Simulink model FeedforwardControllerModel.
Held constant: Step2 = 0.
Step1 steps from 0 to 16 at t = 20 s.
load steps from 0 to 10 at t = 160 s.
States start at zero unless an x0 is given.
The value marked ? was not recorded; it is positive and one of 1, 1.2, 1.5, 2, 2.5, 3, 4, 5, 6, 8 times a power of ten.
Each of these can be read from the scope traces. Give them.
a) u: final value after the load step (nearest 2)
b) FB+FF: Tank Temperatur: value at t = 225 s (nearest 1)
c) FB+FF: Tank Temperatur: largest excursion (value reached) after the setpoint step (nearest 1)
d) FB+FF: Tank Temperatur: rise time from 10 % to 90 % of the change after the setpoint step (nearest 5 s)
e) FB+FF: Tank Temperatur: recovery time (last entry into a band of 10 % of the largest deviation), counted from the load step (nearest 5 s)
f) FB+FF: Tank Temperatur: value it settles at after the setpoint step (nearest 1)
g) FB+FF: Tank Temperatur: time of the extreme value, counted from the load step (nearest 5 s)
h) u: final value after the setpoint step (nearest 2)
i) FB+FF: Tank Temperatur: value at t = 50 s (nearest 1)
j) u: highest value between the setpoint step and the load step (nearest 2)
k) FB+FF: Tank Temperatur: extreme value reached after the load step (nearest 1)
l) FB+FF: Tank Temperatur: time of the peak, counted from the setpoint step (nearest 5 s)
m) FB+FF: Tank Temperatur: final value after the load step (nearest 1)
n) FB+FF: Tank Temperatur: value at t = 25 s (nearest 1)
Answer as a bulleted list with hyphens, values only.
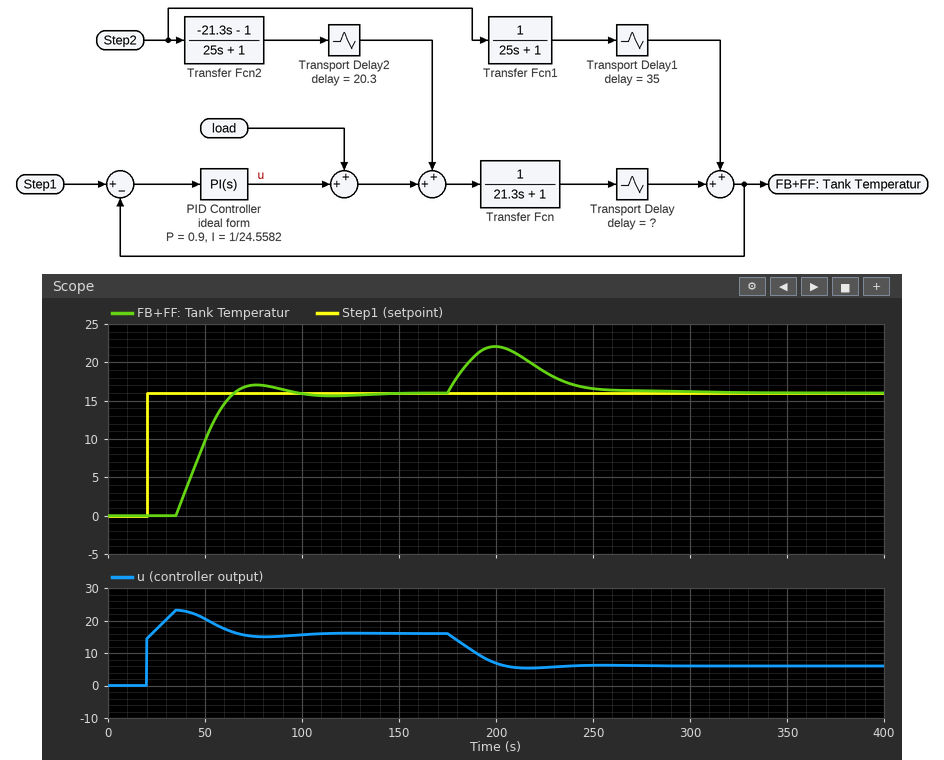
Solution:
- 6
- 19
- 17
- 20 s
- 90 s
- 16
- 40 s
- 16
- 10
- 24
- 22
- 55 s
- 16
- 0
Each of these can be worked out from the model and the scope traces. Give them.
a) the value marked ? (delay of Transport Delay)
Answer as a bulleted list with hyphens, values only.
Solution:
- 15
